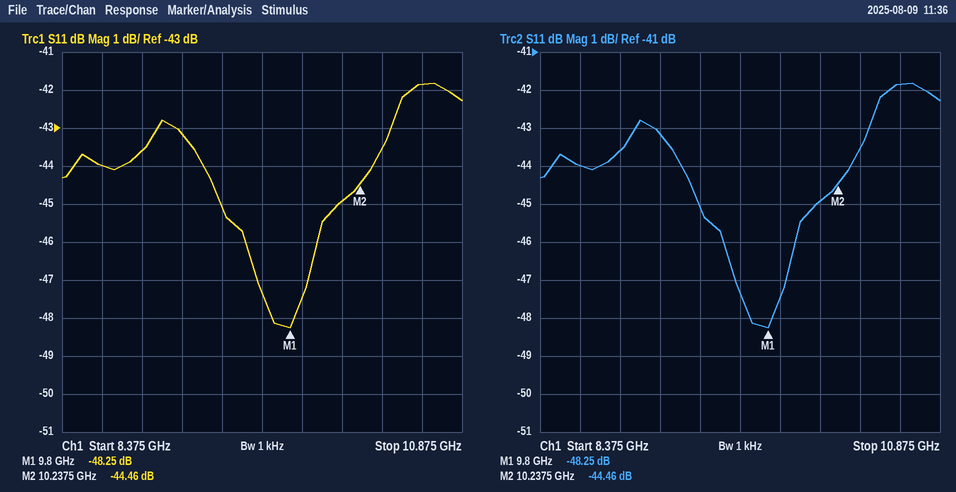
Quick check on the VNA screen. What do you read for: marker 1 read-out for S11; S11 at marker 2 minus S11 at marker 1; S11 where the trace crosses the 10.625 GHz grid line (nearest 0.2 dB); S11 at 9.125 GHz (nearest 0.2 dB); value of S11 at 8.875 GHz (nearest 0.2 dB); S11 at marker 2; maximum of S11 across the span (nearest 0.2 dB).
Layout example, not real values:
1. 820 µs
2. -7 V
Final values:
1. -48.25 dB
2. 3.79 dB
3. -41.8 dB
4. -43.2 dB
5. -43.6 dB
6. -44.46 dB
7. -41.8 dB
